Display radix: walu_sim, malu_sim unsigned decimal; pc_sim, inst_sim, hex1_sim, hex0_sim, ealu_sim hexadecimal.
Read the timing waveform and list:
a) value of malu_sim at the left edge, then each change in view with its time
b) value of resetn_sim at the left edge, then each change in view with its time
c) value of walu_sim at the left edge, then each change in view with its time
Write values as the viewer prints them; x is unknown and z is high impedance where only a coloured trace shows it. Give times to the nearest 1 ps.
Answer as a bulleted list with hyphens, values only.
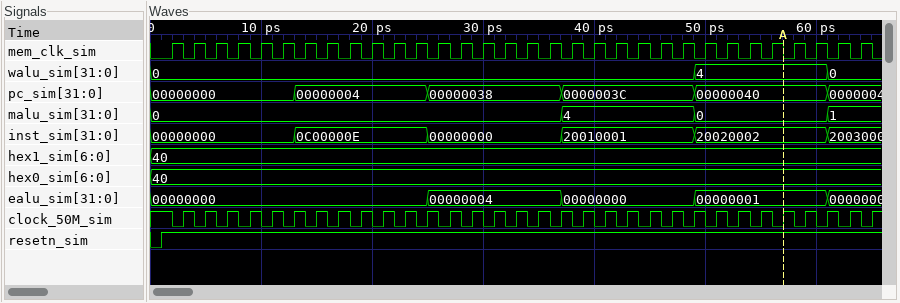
- 0, 4 at 37 ps, 0 at 49 ps, 1 at 61 ps
- 0, 1 at 1 ps
- 0, 4 at 49 ps, 0 at 61 ps
